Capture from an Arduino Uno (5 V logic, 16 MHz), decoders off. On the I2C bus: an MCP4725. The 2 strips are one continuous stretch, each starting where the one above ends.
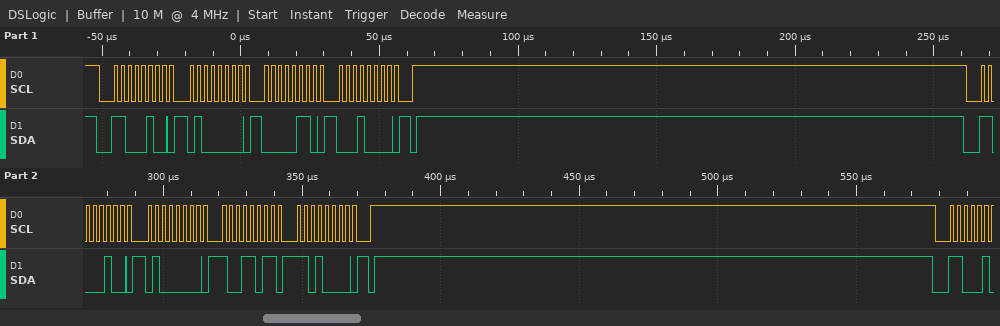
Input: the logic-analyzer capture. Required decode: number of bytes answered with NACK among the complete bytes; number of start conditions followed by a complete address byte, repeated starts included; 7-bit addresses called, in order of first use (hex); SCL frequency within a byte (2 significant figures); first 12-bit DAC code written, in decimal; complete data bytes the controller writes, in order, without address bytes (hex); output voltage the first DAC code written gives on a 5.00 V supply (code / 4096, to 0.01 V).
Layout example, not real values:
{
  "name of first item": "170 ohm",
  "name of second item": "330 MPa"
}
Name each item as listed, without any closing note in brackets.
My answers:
{
  "number of bytes answered with NACK among the complete bytes": "0",
  "number of start conditions followed by a complete address byte, repeated starts included": "2",
  "7-bit addresses called, in order of first use": "0x62",
  "SCL frequency within a byte": "400 kHz",
  "first 12-bit DAC code written, in decimal": "97",
  "complete data bytes the controller writes, in order, without address bytes": "40 06 10 40 9B D0",
  "output voltage the first DAC code written gives on a 5.00 V supply": "0.12 V"
}
